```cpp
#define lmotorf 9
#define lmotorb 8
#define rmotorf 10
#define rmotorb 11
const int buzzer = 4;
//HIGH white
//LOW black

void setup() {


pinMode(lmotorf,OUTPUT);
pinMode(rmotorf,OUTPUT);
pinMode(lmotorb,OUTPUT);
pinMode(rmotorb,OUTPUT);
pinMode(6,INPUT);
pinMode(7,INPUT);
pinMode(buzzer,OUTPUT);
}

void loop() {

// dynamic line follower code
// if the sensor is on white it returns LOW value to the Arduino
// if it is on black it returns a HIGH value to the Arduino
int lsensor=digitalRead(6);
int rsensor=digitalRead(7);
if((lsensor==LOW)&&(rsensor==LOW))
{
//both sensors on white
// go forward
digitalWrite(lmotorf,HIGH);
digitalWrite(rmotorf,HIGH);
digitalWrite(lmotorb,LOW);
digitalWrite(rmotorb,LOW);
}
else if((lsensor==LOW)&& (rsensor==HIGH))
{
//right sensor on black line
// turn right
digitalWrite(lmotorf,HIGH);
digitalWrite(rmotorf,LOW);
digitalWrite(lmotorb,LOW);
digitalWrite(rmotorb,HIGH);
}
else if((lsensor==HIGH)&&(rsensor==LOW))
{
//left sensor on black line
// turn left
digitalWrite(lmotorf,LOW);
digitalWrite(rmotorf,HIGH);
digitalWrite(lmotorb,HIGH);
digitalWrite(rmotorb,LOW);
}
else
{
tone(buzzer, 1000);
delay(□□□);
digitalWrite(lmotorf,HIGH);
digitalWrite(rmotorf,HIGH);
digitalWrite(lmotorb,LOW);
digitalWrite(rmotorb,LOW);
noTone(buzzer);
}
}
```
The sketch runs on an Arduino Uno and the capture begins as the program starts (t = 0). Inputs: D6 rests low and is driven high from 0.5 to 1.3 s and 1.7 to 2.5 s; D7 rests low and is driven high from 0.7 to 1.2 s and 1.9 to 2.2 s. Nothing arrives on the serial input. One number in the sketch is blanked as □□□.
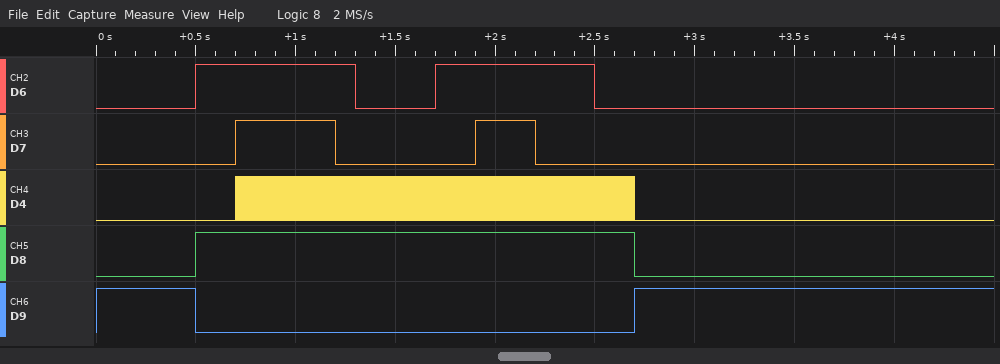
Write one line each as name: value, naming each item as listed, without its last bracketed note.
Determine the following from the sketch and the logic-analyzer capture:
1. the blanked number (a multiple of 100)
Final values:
the blanked number: 2000
